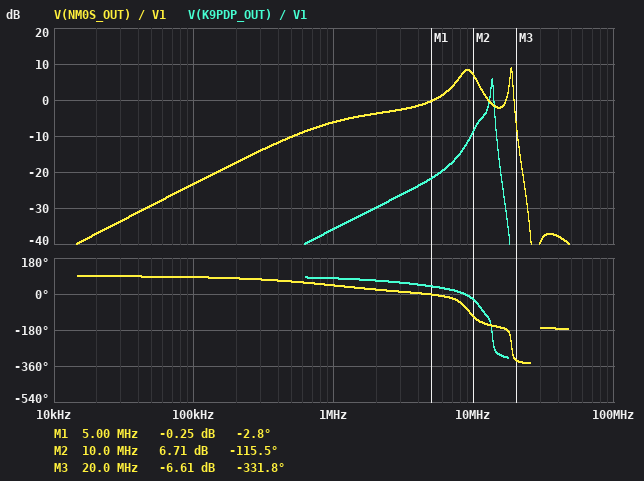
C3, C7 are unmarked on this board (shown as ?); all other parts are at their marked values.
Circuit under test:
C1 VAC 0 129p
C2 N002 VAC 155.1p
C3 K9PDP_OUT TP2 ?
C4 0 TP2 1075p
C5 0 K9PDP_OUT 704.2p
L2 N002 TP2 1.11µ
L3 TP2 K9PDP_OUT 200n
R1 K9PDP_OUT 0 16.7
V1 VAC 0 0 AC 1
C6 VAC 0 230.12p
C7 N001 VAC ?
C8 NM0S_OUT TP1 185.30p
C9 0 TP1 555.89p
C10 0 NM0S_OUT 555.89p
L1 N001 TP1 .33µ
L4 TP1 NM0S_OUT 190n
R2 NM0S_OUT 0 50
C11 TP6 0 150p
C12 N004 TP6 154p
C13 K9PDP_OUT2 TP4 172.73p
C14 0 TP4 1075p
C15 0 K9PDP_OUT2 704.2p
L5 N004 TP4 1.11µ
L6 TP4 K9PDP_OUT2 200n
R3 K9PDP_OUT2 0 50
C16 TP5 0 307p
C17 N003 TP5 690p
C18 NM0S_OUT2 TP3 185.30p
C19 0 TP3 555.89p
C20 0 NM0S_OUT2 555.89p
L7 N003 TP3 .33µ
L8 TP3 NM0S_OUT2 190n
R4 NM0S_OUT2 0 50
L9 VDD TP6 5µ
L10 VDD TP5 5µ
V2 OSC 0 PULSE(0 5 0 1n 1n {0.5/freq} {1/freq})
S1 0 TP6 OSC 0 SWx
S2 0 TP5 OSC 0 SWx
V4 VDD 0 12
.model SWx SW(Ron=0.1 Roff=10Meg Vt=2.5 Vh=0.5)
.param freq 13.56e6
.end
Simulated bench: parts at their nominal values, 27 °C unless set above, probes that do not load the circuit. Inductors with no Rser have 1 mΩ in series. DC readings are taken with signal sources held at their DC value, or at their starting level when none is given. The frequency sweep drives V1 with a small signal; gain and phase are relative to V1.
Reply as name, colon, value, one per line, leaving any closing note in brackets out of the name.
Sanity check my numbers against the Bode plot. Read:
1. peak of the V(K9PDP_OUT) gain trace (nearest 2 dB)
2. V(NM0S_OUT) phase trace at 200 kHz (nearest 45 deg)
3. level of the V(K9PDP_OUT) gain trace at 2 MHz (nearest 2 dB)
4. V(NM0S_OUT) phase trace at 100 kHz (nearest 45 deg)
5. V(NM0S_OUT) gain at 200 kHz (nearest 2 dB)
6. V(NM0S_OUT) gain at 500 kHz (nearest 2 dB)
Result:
peak of the V(K9PDP_OUT) gain trace: 6 dB
V(NM0S_OUT) phase trace at 200 kHz: 90 deg
level of the V(K9PDP_OUT) gain trace at 2 MHz: -30 dB
V(NM0S_OUT) phase trace at 100 kHz: 90 deg
V(NM0S_OUT) gain at 200 kHz: -18 dB
V(NM0S_OUT) gain at 500 kHz: -10 dB
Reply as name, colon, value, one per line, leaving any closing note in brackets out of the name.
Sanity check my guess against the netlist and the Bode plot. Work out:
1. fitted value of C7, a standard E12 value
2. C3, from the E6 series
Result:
fitted value of C7, a standard E12 value: 2.2 nF
C3, from the E6 series: 330 pF
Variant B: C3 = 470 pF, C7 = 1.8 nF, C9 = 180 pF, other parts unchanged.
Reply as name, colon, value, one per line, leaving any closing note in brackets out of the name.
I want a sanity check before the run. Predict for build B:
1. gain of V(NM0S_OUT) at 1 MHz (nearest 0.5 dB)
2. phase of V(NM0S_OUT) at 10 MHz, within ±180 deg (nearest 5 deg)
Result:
gain of V(NM0S_OUT) at 1 MHz: -7.0 dB
phase of V(NM0S_OUT) at 10 MHz, within ±180 deg: -85 deg
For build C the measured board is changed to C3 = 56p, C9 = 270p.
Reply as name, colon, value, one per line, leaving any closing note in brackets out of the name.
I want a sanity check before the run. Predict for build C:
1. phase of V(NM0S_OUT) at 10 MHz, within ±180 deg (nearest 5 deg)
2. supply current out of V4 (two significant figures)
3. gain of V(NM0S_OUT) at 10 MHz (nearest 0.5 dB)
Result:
phase of V(NM0S_OUT) at 10 MHz, within ±180 deg: -100 deg
supply current out of V4: 2.4 µA
gain of V(NM0S_OUT) at 10 MHz: 6.0 dB
